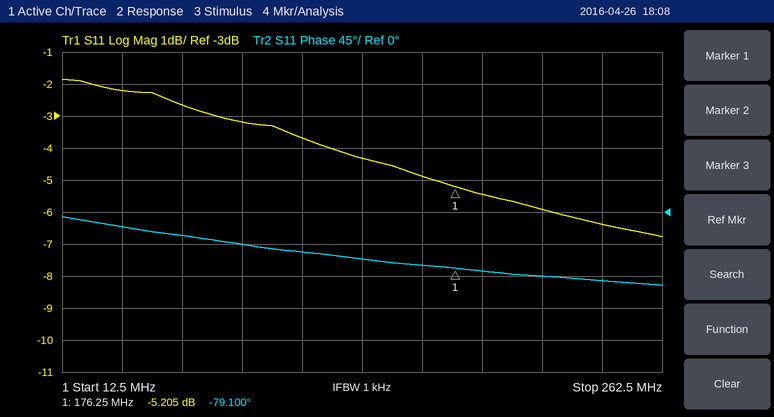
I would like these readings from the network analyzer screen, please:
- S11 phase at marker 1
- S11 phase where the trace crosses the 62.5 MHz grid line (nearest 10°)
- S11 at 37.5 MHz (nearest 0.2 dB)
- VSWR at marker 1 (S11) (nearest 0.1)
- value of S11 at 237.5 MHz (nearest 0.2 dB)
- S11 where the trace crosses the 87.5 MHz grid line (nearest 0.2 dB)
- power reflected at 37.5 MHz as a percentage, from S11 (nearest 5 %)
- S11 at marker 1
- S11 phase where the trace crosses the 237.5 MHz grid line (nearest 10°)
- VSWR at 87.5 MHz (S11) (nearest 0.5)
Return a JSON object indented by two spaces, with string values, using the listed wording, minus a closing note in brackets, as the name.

{
  "S11 phase at marker 1": "-79.100°",
  "S11 phase where the trace crosses the 62.5 MHz grid line": "-30°",
  "S11 at 37.5 MHz": "-2.2 dB",
  "VSWR at marker 1 (S11)": "3.4",
  "value of S11 at 237.5 MHz": "-6.4 dB",
  "S11 where the trace crosses the 87.5 MHz grid line": "-3.2 dB",
  "power reflected at 37.5 MHz as a percentage, from S11": "60 %",
  "S11 at marker 1": "-5.205 dB",
  "S11 phase where the trace crosses the 237.5 MHz grid line": "-100°",
  "VSWR at 87.5 MHz (S11)": "5.5"
}
